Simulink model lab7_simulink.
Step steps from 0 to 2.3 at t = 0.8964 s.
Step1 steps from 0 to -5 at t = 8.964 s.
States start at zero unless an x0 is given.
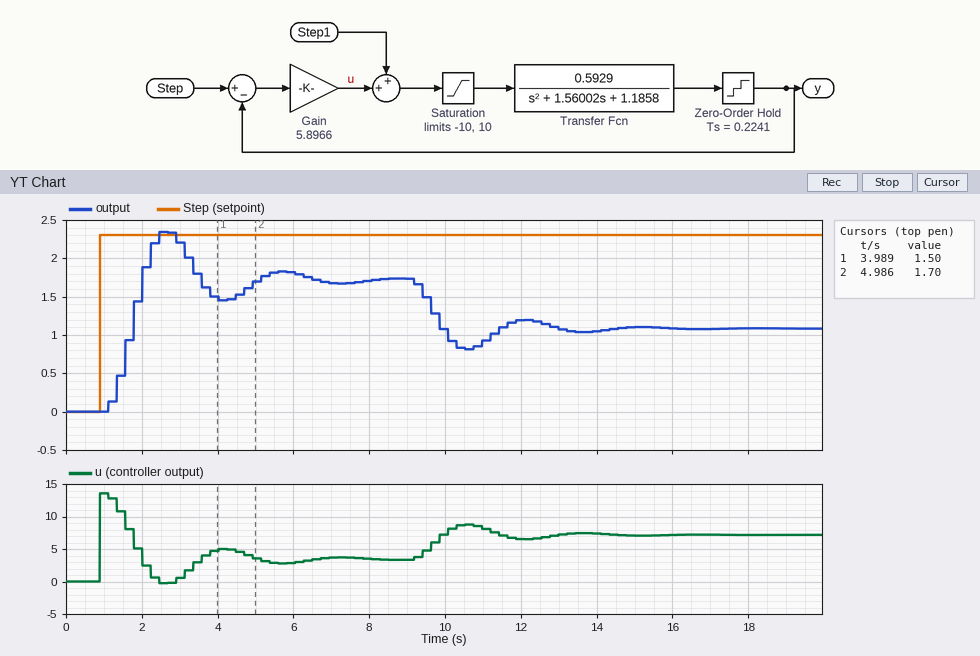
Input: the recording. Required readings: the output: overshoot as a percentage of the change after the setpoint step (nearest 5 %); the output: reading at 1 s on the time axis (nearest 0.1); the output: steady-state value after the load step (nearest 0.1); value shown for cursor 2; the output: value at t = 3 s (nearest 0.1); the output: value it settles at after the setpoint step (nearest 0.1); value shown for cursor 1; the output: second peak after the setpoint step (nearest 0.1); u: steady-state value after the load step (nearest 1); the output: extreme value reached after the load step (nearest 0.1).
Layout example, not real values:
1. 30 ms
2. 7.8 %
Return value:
1. 35 %
2. 0.0
3. 1.1
4. 1.70
5. 2.2
6. 1.7
7. 1.50
8. 1.8
9. 7
10. 0.8
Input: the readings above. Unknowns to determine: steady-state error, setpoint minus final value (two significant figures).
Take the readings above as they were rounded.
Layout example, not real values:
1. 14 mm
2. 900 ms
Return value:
1. 0.60
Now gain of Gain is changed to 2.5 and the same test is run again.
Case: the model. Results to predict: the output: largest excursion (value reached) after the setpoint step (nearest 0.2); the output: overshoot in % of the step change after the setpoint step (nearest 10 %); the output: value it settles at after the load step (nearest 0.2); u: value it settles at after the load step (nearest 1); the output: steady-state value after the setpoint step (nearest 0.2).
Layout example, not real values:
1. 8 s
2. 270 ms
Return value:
1. 1.6
2. 20 %
3. 0.2
4. 5
5. 1.2
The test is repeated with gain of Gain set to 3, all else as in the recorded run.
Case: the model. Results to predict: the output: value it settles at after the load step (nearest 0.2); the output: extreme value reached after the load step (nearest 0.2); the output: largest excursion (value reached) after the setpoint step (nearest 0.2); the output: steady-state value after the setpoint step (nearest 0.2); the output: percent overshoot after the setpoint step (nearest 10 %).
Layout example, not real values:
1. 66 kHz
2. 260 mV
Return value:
1. 0.4
2. 0.2
3. 1.8
4. 1.4
5. 30 %
